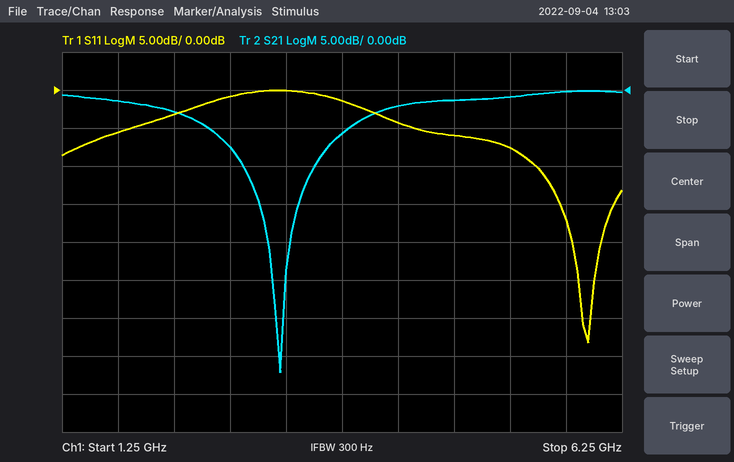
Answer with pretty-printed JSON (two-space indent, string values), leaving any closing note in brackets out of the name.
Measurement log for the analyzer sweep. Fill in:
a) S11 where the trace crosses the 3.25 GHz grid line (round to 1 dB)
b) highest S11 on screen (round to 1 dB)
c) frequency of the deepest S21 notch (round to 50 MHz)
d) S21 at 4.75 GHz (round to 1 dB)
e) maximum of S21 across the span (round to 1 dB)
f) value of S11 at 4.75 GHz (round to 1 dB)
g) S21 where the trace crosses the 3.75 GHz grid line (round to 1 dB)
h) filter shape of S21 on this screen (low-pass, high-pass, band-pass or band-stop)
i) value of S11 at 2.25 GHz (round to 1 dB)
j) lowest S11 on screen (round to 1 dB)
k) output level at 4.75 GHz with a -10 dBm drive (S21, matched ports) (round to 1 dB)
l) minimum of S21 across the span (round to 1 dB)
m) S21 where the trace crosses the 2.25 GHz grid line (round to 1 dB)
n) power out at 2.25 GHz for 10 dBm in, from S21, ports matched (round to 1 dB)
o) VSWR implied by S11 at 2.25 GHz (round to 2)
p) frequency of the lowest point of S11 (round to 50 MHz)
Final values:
{
  "S11 where the trace crosses the 3.25 GHz grid line": "0 dB",
  "highest S11 on screen": "0 dB",
  "frequency of the deepest S21 notch": "3.20 GHz",
  "S21 at 4.75 GHz": "-1 dB",
  "maximum of S21 across the span": "0 dB",
  "value of S11 at 4.75 GHz": "-6 dB",
  "S21 where the trace crosses the 3.75 GHz grid line": "-6 dB",
  "filter shape of S21 on this screen": "band-stop",
  "value of S11 at 2.25 GHz": "-3 dB",
  "lowest S11 on screen": "-33 dB",
  "output level at 4.75 GHz with a -10 dBm drive (S21, matched ports)": "-11 dBm",
  "minimum of S21 across the span": "-37 dB",
  "S21 where the trace crosses the 2.25 GHz grid line": "-3 dB",
  "power out at 2.25 GHz for 10 dBm in, from S21, ports matched": "7 dBm",
  "VSWR implied by S11 at 2.25 GHz": "6",
  "frequency of the lowest point of S11": "5.95 GHz"
}
